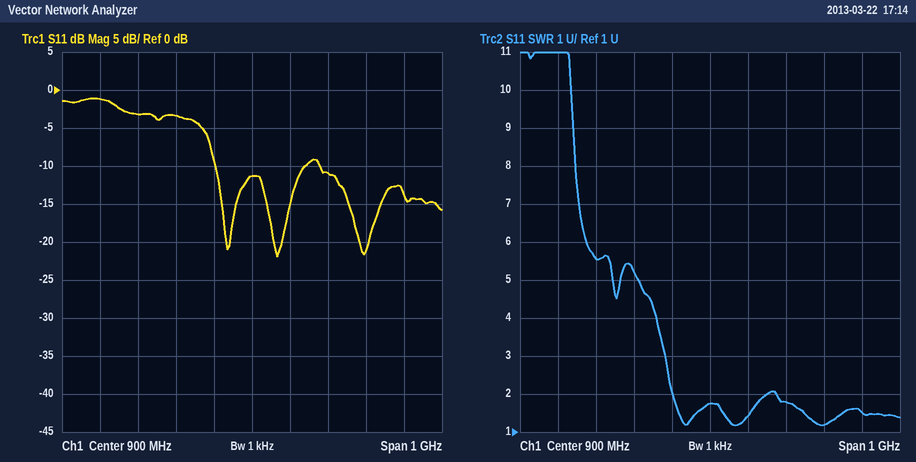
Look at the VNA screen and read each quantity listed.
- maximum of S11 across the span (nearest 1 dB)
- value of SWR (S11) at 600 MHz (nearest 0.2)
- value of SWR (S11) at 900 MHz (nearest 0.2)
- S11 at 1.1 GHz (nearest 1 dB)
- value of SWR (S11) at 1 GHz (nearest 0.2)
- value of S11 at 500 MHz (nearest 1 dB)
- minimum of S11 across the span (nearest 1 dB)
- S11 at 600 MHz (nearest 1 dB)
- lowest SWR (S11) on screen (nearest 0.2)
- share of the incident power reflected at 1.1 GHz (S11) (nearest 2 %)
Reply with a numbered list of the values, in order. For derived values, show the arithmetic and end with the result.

1. -1 dB
2. 5.6
3. 1.8
4. -11 dB
5. 1.4
6. -1 dB
7. -22 dB
8. -3 dB
9. 1.2
10. 10^(-11/10) ≈ 8 %
